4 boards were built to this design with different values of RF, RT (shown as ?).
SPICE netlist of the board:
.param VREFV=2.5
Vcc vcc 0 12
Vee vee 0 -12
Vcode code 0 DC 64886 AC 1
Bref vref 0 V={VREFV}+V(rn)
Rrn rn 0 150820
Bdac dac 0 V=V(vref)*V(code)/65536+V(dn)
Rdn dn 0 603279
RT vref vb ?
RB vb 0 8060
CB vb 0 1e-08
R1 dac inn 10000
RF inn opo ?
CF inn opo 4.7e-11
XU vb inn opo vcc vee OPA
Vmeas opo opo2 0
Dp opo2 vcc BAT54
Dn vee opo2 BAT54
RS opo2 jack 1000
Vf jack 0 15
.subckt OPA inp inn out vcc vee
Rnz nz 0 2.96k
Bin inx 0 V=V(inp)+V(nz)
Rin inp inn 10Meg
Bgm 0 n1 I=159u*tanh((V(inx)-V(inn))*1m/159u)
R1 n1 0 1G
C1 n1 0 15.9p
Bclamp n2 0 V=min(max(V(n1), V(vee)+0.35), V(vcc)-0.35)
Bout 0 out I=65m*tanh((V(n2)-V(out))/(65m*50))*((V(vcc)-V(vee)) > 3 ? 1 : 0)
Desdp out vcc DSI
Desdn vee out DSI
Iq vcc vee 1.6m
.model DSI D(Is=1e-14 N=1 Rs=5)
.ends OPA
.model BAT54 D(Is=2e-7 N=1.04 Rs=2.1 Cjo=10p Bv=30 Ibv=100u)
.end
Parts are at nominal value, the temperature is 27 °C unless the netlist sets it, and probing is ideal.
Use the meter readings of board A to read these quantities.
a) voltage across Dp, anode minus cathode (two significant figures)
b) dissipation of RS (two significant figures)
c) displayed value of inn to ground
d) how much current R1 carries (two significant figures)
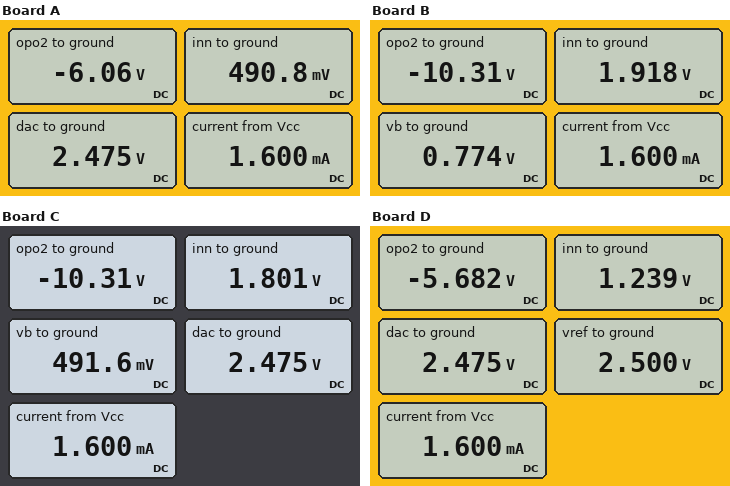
-18 V
440 mW
490.8 mV
200 µA
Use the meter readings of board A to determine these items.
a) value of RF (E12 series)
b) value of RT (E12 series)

33 kΩ
33 kΩ
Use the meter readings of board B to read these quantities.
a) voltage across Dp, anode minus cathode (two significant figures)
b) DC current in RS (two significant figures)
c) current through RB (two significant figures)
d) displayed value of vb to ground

-22 V
25 mA
96 µA
0.774 V
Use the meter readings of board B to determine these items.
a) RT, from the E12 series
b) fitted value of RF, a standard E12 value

18 kΩ
220 kΩ
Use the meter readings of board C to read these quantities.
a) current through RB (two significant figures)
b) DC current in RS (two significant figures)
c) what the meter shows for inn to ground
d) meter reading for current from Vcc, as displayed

61 µA
25 mA
1.801 V
1.600 mA
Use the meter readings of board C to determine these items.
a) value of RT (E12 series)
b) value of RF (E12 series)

33 kΩ
180 kΩ
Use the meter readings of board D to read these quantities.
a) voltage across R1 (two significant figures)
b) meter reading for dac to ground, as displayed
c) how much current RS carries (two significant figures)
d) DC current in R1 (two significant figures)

1.2 V
2.475 V
21 mA
120 µA
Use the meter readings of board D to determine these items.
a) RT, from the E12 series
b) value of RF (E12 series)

8.2 kΩ
56 kΩ
